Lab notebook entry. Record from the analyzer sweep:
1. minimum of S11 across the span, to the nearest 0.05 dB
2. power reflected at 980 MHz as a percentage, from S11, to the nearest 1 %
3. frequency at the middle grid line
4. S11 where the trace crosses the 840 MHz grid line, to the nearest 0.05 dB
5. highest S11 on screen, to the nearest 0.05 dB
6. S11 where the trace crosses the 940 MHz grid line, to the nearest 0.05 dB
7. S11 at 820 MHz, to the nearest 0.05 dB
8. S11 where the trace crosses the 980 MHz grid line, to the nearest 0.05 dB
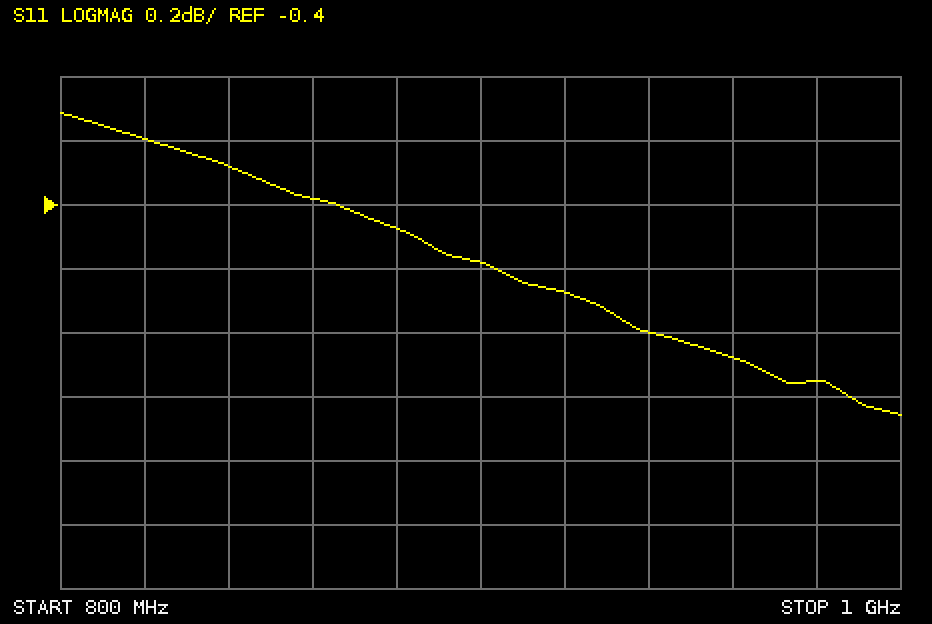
-1.05 dB
80 %
900 MHz
-0.30 dB
-0.10 dB
-0.80 dB
-0.20 dB
-0.95 dB
